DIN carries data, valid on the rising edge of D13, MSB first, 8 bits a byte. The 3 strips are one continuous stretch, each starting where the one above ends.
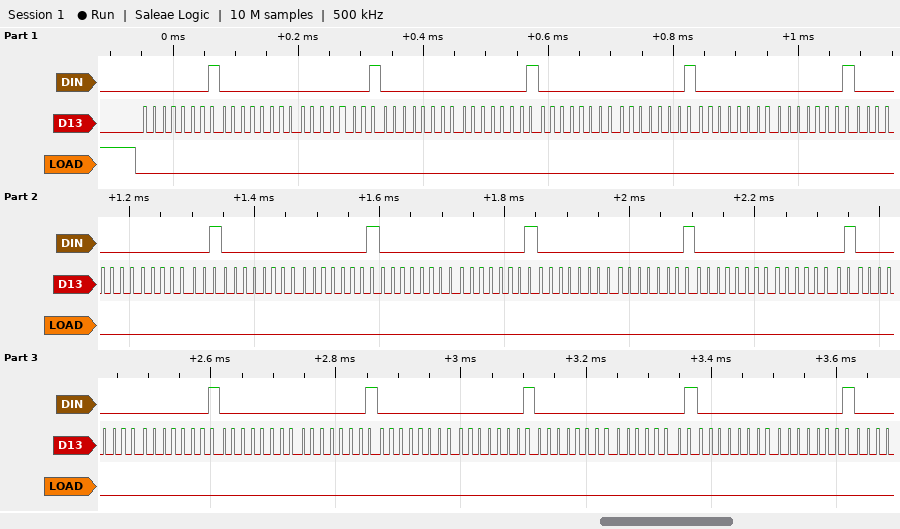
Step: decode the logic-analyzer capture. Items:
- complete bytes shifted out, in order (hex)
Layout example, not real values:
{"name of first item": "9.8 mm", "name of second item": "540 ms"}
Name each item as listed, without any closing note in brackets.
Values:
{"complete bytes shifted out, in order": "01 00 01 00 01 00 01 00 01 00 01 00 01 00 01 00 01 00 01 00 01 00 01 00 01 00 01 00 01"}
